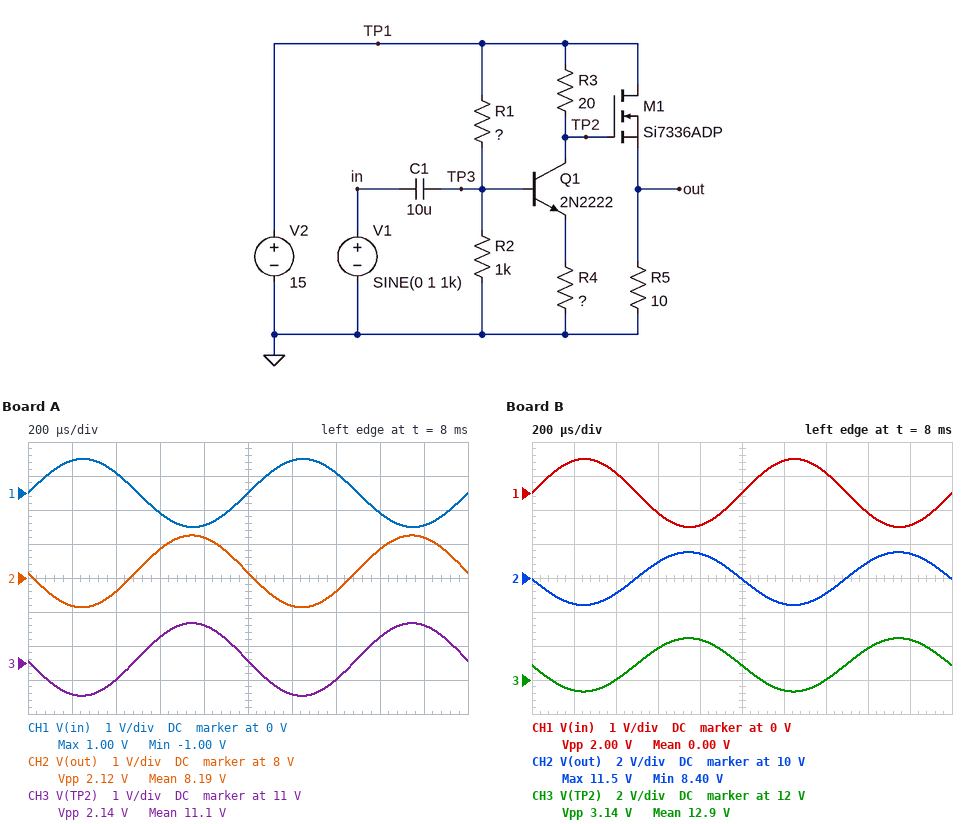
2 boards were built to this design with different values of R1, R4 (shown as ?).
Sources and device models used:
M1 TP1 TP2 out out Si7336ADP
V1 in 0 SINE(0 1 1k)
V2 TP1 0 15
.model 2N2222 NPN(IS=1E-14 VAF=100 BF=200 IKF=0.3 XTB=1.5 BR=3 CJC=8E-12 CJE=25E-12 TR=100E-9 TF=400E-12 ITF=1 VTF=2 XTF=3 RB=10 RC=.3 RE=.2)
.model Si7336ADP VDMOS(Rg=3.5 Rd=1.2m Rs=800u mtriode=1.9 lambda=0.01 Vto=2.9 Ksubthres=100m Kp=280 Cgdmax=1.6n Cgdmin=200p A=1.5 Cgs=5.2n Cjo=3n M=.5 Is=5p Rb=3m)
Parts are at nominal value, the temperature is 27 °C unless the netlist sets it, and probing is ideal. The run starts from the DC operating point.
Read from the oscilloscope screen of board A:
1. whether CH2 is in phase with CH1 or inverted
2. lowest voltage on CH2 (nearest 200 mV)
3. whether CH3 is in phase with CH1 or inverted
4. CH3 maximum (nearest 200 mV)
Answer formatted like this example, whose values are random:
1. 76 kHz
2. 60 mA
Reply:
1. inverted
2. 7.2 V
3. inverted
4. 12.2 V
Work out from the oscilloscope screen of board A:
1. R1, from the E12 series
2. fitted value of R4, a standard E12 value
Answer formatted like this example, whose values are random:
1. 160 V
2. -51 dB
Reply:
1. 1.8 kΩ
2. 18 Ω
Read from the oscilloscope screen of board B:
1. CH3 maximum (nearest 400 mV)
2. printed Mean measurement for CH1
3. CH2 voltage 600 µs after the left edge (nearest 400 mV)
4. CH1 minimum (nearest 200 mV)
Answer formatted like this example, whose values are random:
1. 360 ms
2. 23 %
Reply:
1. 14.4 V
2. 0.00 V
3. 10.8 V
4. -1.0 V
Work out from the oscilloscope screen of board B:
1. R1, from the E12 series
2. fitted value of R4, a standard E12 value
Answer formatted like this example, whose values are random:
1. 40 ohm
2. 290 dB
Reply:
1. 4.7 kΩ
2. 12 Ω
